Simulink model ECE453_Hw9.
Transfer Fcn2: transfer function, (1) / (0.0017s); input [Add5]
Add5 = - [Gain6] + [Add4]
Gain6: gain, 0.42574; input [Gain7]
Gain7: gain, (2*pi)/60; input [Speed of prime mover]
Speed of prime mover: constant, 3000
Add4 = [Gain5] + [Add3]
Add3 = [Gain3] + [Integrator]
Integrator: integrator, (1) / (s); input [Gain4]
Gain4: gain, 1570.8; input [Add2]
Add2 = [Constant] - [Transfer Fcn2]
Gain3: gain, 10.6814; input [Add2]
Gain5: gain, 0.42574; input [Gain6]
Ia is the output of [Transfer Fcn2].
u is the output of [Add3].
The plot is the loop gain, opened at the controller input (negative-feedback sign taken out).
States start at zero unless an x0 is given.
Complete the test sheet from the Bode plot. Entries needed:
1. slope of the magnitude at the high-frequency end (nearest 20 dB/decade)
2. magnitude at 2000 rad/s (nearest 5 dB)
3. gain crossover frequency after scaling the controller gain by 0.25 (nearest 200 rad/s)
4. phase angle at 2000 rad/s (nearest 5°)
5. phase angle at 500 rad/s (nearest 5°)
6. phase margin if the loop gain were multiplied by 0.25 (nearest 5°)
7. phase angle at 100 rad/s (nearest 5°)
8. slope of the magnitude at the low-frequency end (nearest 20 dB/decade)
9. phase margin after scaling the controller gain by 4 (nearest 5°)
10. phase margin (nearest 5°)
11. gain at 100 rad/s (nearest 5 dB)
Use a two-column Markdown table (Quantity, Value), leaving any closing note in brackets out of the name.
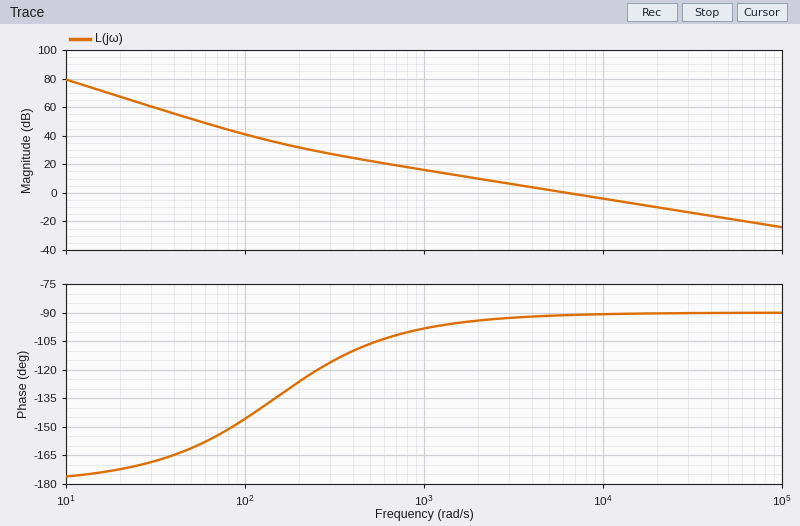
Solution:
| Quantity | Value |
|---|---|
| slope of the magnitude at the high-frequency end | -20 dB/decade |
| magnitude at 2000 rad/s | 10 dB |
| gain crossover frequency after scaling the controller gain by 0.25 | 1600 rad/s |
| phase angle at 2000 rad/s | -95° |
| phase angle at 500 rad/s | -105° |
| phase margin if the loop gain were multiplied by 0.25 | 85° |
| phase angle at 100 rad/s | -145° |
| slope of the magnitude at the low-frequency end | -40 dB/decade |
| phase margin after scaling the controller gain by 4 | 90° |
| phase margin | 90° |
| gain at 100 rad/s | 40 dB |
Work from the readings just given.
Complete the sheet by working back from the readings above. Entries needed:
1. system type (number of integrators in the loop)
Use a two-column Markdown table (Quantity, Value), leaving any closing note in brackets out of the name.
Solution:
| Quantity | Value |
|---|---|
| system type | 2 |
